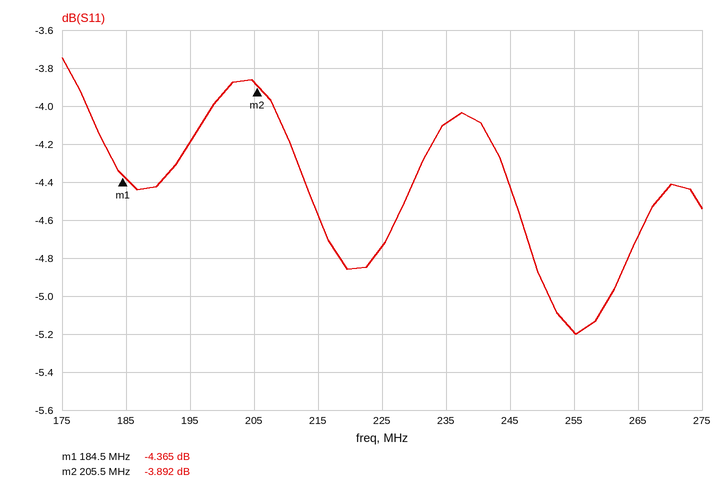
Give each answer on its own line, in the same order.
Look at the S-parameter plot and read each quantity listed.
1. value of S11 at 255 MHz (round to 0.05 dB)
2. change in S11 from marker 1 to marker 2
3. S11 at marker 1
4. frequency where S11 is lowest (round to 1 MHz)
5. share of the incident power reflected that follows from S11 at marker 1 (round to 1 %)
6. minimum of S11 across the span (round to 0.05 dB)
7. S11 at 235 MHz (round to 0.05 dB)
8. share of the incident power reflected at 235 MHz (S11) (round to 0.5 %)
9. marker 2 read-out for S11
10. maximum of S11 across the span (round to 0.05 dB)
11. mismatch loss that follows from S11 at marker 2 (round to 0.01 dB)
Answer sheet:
-5.20 dB
0.473 dB
-4.365 dB
255 MHz
37 %
-5.20 dB
-4.10 dB
39.0 %
-3.892 dB
-3.75 dB
2.28 dB
